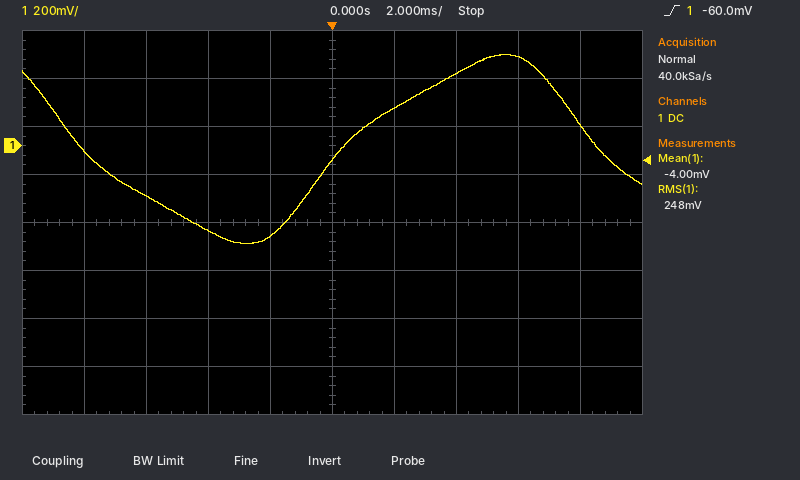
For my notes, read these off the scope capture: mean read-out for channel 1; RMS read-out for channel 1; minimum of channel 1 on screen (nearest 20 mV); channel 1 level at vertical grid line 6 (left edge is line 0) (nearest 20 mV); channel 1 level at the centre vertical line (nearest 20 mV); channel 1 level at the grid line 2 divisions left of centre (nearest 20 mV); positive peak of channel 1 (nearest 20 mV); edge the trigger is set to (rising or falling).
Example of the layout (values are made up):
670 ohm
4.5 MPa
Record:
-4.00 mV
248 mV
-400 mV
160 mV
-60 mV
-360 mV
380 mV
rising
